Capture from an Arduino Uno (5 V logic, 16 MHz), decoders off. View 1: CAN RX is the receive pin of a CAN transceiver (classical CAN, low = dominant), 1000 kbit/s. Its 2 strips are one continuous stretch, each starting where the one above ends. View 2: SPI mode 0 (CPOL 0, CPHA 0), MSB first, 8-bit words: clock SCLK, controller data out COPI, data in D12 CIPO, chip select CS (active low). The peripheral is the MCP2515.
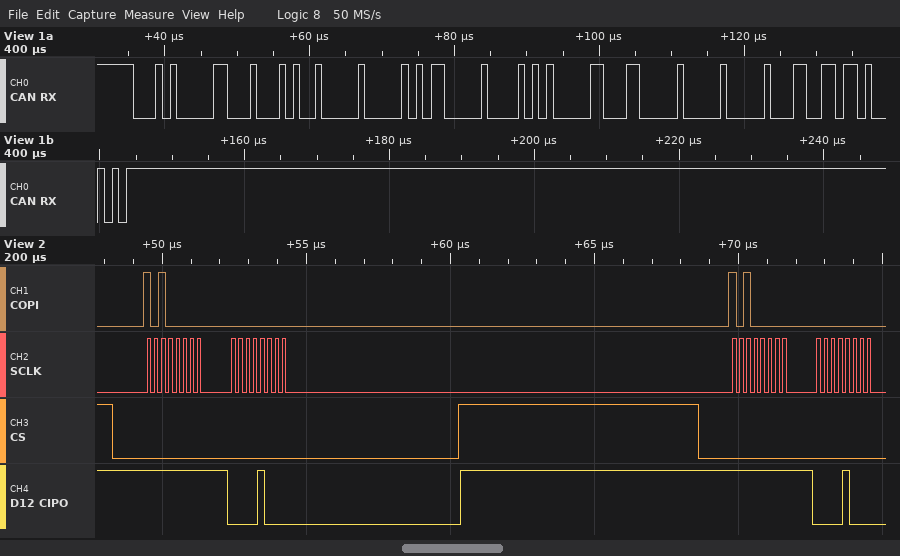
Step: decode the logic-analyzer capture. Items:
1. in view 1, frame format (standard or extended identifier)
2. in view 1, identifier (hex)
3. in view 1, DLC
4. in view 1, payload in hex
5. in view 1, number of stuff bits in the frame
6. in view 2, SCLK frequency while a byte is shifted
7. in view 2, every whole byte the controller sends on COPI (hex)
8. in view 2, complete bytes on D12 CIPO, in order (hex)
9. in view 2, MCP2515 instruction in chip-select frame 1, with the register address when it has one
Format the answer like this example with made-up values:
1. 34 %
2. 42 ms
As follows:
1. standard
2. 0x141
3. 8
4. A4 00 58 02 A0 8C 00 00
5. 8
6. 4 MHz
7. A0 00 A0 00
8. FF 08 FF 08
9. READ STATUS
